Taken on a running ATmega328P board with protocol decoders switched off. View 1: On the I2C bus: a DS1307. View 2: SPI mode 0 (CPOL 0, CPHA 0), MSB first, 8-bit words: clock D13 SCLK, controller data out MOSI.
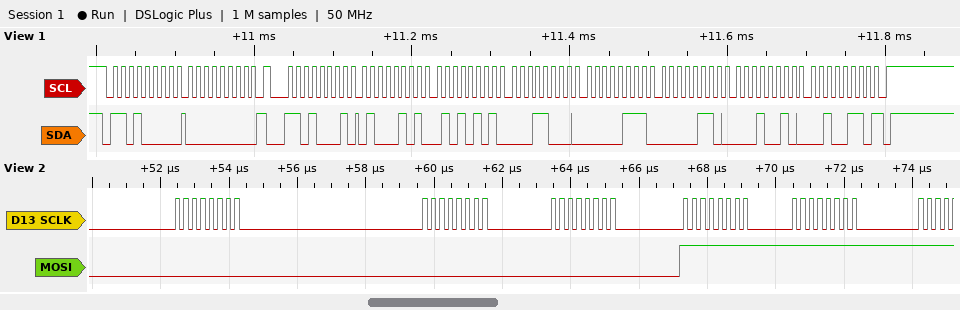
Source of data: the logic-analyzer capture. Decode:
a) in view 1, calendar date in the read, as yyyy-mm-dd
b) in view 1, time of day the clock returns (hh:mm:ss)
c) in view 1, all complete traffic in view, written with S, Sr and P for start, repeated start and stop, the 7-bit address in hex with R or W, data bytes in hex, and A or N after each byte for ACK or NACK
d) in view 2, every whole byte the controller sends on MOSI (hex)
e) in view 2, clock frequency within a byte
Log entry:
2026-12-06
18:55:45
S 68W A 00 A Sr 68R A 45 A 55 A 18 A 07 A 06 A 12 A 26 N P
00 00 00 FF FF
4 MHz
